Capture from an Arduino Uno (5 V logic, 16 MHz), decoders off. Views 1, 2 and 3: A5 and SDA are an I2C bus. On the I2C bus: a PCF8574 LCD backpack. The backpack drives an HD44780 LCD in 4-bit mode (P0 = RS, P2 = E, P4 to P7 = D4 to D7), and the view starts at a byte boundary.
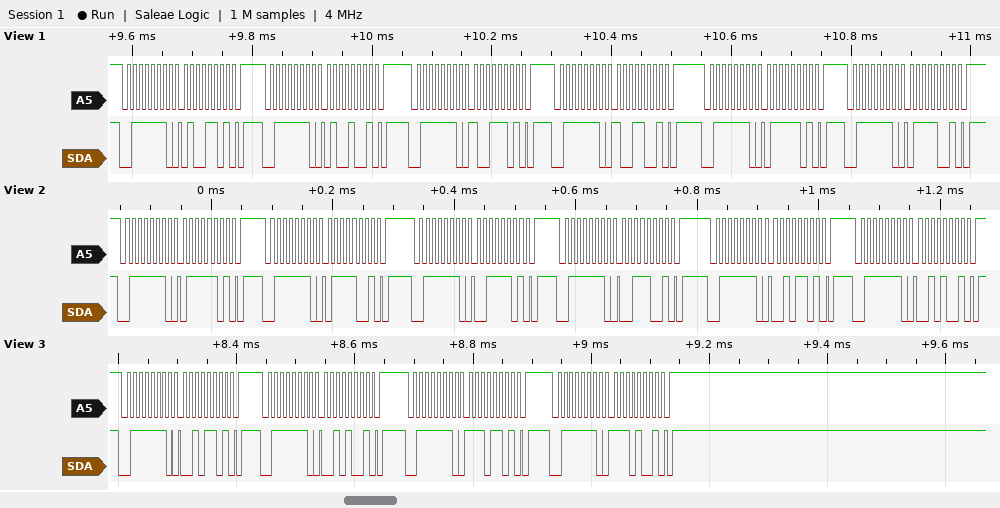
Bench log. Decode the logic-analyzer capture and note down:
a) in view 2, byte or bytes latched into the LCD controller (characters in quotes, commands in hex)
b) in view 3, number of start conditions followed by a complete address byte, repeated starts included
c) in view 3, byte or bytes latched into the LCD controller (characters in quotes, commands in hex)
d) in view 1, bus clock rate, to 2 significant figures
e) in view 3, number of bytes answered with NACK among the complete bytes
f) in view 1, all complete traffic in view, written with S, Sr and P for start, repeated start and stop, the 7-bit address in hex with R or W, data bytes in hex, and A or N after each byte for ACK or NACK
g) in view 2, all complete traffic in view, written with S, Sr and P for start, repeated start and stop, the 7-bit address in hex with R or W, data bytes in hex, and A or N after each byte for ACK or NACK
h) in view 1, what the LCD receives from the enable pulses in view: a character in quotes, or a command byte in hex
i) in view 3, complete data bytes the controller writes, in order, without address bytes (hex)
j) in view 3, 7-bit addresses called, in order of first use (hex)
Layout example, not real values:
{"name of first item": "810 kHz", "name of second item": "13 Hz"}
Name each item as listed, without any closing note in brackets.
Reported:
{"in view 2, byte or bytes latched into the LCD controller": "'s'", "in view 3, number of start conditions followed by a complete address byte, repeated starts included": "4", "in view 3, byte or bytes latched into the LCD controller": "'.'", "in view 1, bus clock rate, to 2 significant figures": "100 kHz", "in view 3, number of bytes answered with NACK among the complete bytes": "0", "in view 1, all complete traffic in view, written with S, Sr and P for start, repeated start and stop, the 7-bit address in hex with R or W, data bytes in hex, and A or N after each byte for ACK or NACK": "S 3FW A 4D A P S 3FW A 49 A P S 3FW A 9D A P S 3FW A 99 A P S 3FW A 7D A P S 3FW A 79 A P", "in view 2, all complete traffic in view, written with S, Sr and P for start, repeated start and stop, the 7-bit address in hex with R or W, data bytes in hex, and A or N after each byte for ACK or NACK": "S 3FW A 7D A P S 3FW A 79 A P S 3FW A 3D A P S 3FW A 39 A P S 3FW A 2D A P S 3FW A 29 A P", "in view 1, what the LCD receives from the enable pulses in view: a character in quotes, or a command byte in hex": "'I'", "in view 3, complete data bytes the controller writes, in order, without address bytes": "2D 29 ED E9", "in view 3, 7-bit addresses called, in order of first use": "0x3F"}
